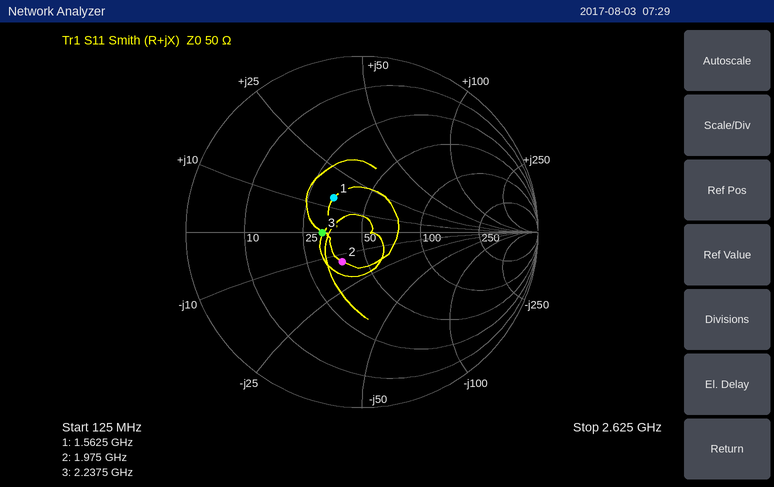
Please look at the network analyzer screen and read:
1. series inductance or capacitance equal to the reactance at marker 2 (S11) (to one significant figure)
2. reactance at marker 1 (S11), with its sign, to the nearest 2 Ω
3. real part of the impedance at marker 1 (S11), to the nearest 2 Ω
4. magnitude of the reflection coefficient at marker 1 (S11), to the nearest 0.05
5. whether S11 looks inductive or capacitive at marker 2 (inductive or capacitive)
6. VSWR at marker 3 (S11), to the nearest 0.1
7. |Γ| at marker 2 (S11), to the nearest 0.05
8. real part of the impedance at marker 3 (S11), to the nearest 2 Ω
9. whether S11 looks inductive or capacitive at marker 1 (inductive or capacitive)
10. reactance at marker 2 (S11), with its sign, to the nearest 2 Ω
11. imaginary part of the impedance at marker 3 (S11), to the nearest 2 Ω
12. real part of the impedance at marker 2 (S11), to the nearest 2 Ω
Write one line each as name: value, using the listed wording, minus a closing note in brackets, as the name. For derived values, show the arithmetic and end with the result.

series inductance or capacitance equal to the reactance at marker 2 (S11): C = 1/(2π × 1.975 GHz × 14 Ω) ≈ 6 pF
reactance at marker 1 (S11), with its sign, to the nearest 2 Ω: +14 Ω
real part of the impedance at marker 1 (S11), to the nearest 2 Ω: 34 Ω
magnitude of the reflection coefficient at marker 1 (S11), to the nearest 0.05: 0.25
whether S11 looks inductive or capacitive at marker 2: capacitive
VSWR at marker 3 (S11), to the nearest 0.1: 1.6
|Γ| at marker 2 (S11), to the nearest 0.05: 0.20
real part of the impedance at marker 3 (S11), to the nearest 2 Ω: 32 Ω
whether S11 looks inductive or capacitive at marker 1: inductive
reactance at marker 2 (S11), with its sign, to the nearest 2 Ω: -14 Ω
imaginary part of the impedance at marker 3 (S11), to the nearest 2 Ω: 0 Ω
real part of the impedance at marker 2 (S11), to the nearest 2 Ω: 38 Ω
